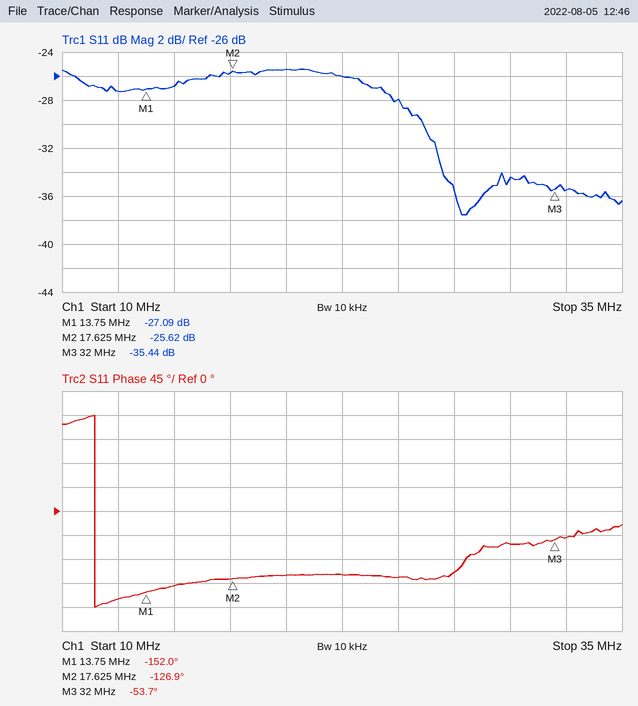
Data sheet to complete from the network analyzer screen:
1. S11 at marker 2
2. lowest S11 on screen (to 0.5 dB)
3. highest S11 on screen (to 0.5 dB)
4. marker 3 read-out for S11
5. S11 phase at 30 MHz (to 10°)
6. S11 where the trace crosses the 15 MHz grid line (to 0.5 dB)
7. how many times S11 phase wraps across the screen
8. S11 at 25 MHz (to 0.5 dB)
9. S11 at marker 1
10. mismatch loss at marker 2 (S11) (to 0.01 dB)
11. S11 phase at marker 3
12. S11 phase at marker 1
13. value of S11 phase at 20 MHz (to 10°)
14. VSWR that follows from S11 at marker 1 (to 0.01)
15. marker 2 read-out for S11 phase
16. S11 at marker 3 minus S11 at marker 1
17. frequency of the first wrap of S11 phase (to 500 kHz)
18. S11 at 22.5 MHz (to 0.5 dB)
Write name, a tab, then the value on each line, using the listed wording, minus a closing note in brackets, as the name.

S11 at marker 2	-25.62 dB
lowest S11 on screen	-37.5 dB
highest S11 on screen	-25.5 dB
marker 3 read-out for S11	-35.44 dB
S11 phase at 30 MHz	-60°
S11 where the trace crosses the 15 MHz grid line	-27.0 dB
how many times S11 phase wraps across the screen	1
S11 at 25 MHz	-28.0 dB
S11 at marker 1	-27.09 dB
mismatch loss at marker 2 (S11)	0.01 dB
S11 phase at marker 3	-53.7°
S11 phase at marker 1	-152.0°
value of S11 phase at 20 MHz	-120°
VSWR that follows from S11 at marker 1	1.09
marker 2 read-out for S11 phase	-126.9°
S11 at marker 3 minus S11 at marker 1	-8.35 dB
frequency of the first wrap of S11 phase	11.5 MHz
S11 at 22.5 MHz	-26.0 dB
